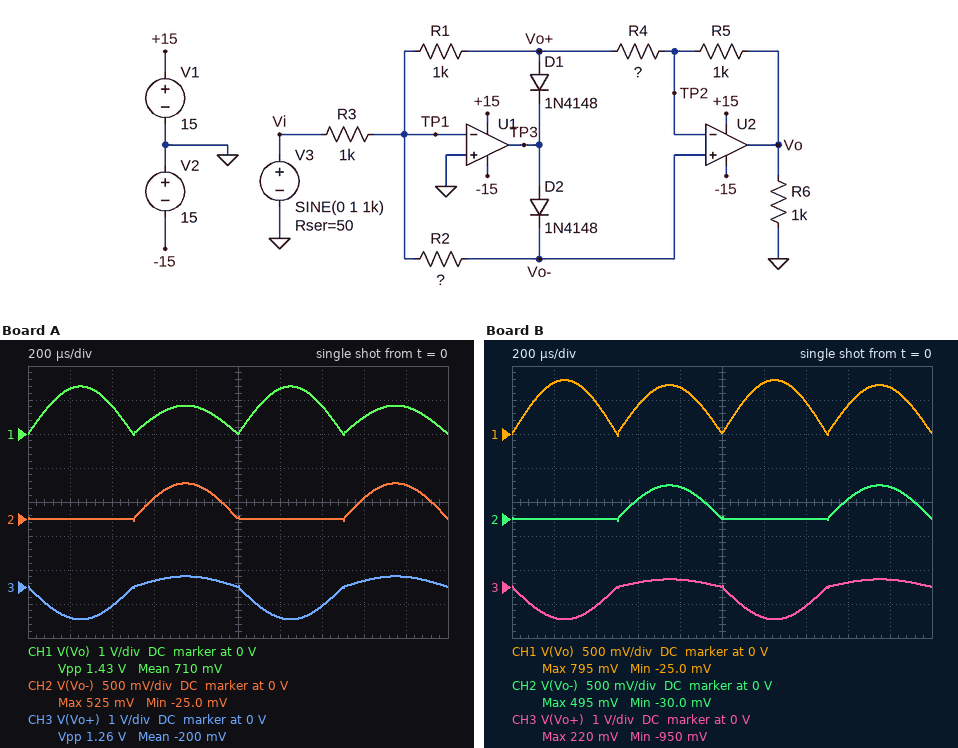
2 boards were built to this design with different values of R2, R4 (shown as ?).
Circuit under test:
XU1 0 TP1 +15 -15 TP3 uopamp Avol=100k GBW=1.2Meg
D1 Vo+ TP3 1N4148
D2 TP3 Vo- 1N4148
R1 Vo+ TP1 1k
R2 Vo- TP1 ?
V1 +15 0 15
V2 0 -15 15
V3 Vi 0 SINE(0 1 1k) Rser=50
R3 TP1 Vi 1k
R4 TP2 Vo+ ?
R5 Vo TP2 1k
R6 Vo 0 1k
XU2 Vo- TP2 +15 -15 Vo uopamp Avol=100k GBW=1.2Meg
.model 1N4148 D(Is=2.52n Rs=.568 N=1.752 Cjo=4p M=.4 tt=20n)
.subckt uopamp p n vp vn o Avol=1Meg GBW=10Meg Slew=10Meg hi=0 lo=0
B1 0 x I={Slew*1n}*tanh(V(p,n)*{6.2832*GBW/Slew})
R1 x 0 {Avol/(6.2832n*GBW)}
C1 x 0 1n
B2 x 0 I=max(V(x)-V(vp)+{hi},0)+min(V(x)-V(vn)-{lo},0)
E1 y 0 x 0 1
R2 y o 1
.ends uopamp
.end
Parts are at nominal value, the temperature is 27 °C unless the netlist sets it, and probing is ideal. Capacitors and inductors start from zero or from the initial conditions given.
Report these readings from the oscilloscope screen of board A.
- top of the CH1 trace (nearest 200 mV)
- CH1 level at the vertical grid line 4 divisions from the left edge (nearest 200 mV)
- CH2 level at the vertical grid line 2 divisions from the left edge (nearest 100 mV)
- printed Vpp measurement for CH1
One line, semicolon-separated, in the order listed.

1.4 V; 800 mV; 0 V; 1.43 V
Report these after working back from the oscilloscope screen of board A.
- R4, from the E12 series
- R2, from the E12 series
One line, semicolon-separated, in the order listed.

680 Ω; 820 Ω
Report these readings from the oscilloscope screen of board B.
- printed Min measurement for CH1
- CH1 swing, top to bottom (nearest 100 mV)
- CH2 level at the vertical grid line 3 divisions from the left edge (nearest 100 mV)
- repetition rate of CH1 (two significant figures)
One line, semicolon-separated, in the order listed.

-25.0 mV; 800 mV; 300 mV; 2.0 kHz
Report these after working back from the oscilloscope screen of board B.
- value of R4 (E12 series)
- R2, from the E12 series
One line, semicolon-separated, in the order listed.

1.2 kΩ; 680 Ω
